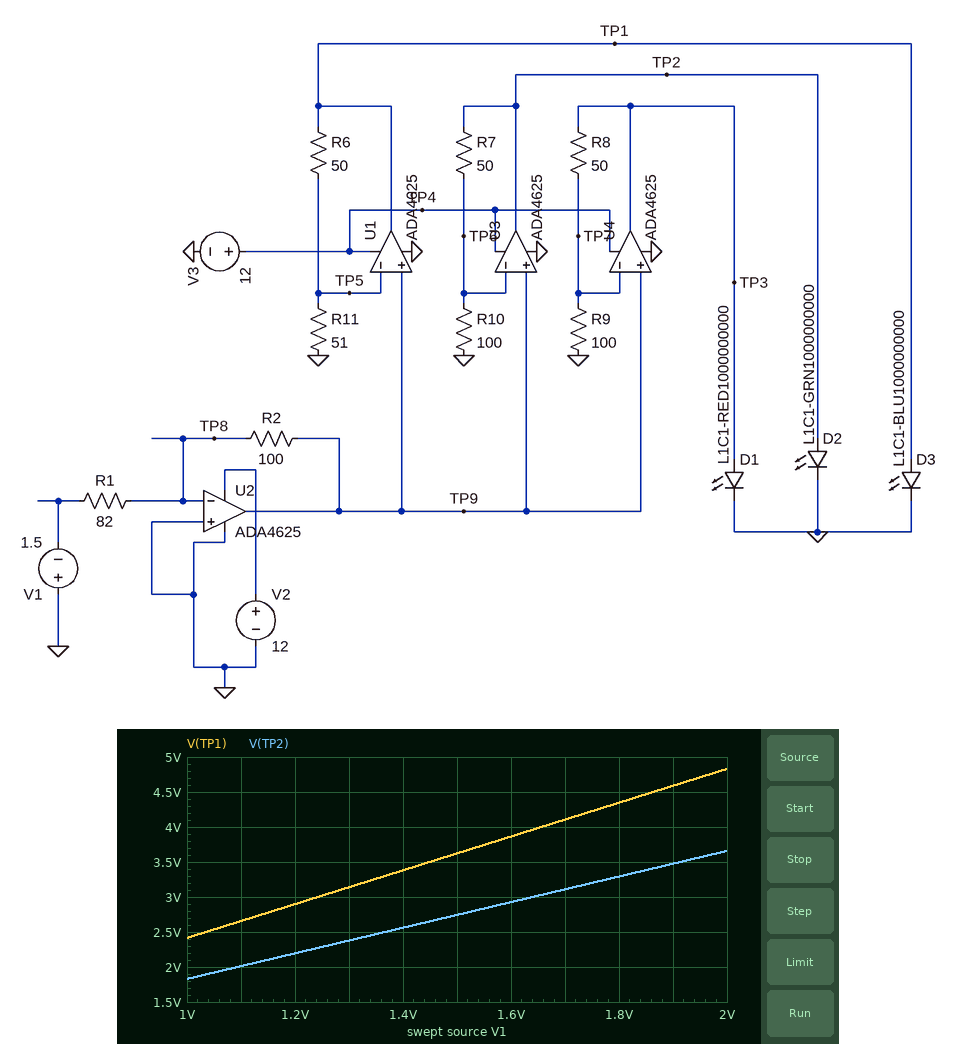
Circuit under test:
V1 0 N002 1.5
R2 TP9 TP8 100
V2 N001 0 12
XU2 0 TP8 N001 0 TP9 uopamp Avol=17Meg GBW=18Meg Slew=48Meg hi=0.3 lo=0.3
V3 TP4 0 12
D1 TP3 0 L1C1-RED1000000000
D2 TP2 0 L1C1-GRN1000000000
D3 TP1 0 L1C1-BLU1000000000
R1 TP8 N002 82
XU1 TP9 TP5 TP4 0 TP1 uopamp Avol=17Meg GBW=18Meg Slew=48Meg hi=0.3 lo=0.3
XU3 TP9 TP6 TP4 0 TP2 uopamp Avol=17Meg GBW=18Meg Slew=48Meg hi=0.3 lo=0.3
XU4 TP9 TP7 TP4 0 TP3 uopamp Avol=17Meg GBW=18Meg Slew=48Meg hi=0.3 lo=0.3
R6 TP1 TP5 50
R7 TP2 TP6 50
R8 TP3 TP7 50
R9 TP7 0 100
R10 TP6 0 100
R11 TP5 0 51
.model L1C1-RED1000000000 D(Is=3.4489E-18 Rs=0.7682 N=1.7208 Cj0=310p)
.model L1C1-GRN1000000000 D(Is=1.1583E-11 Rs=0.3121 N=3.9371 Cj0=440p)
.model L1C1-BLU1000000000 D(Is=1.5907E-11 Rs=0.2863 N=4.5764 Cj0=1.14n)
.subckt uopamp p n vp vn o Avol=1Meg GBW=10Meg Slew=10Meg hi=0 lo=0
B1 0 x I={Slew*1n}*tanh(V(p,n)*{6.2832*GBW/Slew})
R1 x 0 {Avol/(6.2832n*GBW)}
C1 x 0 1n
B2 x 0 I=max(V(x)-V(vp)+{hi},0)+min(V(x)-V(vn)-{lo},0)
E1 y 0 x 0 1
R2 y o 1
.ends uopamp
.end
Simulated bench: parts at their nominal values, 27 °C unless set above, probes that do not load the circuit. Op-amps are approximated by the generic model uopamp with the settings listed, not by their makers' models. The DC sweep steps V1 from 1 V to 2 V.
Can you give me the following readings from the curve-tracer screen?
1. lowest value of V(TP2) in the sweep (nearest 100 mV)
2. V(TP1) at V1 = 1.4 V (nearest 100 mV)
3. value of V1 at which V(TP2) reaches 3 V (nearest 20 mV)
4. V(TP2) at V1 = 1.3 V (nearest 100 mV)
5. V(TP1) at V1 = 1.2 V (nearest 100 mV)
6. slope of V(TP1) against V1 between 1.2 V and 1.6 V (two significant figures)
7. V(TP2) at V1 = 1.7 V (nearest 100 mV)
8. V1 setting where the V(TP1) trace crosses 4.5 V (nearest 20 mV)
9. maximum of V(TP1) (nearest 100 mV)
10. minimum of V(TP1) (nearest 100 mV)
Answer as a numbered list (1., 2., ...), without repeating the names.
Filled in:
1. 1.8 V
2. 3.4 V
3. 1.64 V
4. 2.4 V
5. 2.9 V
6. 2.4 V/V
7. 3.1 V
8. 1.86 V
9. 4.8 V
10. 2.4 V
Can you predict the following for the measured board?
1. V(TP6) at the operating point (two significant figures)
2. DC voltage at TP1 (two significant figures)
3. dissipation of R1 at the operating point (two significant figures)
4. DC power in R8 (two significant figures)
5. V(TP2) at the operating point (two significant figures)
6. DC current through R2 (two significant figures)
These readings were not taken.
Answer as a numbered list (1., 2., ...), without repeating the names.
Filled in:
1. 1.8 V
2. 3.6 V
3. 27 mW
4. 17 mW
5. 2.7 V
6. 18 mA
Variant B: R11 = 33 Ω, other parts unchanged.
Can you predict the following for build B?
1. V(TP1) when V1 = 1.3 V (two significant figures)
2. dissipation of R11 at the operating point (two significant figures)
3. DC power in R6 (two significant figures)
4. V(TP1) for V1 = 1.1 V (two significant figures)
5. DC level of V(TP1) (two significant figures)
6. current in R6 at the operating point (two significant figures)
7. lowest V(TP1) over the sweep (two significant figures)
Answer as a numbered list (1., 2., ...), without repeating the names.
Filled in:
1. 4.0 V
2. 100 mW
3. 150 mW
4. 3.4 V
5. 4.6 V
6. 55 mA
7. 3.1 V
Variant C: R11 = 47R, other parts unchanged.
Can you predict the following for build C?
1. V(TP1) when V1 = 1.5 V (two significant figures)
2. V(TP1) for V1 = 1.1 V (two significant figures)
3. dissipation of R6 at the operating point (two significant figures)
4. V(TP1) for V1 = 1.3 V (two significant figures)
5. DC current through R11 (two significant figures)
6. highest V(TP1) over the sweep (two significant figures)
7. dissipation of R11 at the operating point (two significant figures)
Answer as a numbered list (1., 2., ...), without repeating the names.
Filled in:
1. 3.8 V
2. 2.8 V
3. 76 mW
4. 3.3 V
5. 39 mA
6. 5.0 V
7. 71 mW
